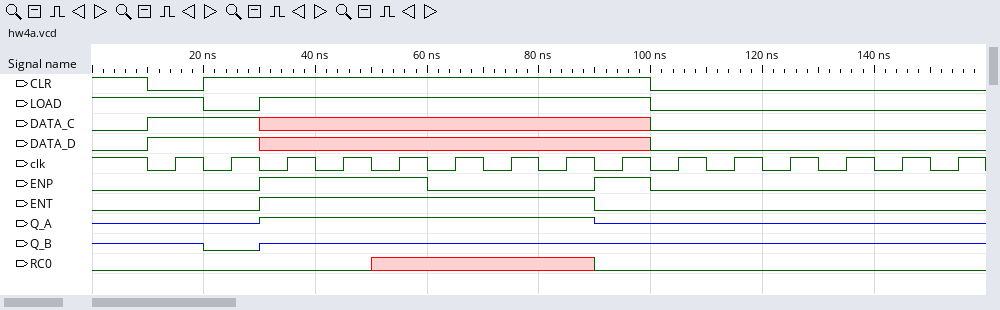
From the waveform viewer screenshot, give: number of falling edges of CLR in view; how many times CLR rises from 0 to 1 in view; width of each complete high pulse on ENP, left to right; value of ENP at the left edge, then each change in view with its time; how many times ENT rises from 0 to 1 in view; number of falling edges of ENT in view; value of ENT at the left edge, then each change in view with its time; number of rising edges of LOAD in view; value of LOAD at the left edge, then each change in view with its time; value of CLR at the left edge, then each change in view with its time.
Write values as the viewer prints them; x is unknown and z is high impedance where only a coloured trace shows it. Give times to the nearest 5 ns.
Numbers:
2
1
30 ns, 10 ns
0, 1 at 30 ns, 0 at 60 ns, 1 at 90 ns, 0 at 100 ns
1
1
0, 1 at 30 ns, 0 at 90 ns
1
1, 0 at 20 ns, 1 at 30 ns, 0 at 100 ns
1, 0 at 10 ns, 1 at 20 ns, 0 at 100 ns
